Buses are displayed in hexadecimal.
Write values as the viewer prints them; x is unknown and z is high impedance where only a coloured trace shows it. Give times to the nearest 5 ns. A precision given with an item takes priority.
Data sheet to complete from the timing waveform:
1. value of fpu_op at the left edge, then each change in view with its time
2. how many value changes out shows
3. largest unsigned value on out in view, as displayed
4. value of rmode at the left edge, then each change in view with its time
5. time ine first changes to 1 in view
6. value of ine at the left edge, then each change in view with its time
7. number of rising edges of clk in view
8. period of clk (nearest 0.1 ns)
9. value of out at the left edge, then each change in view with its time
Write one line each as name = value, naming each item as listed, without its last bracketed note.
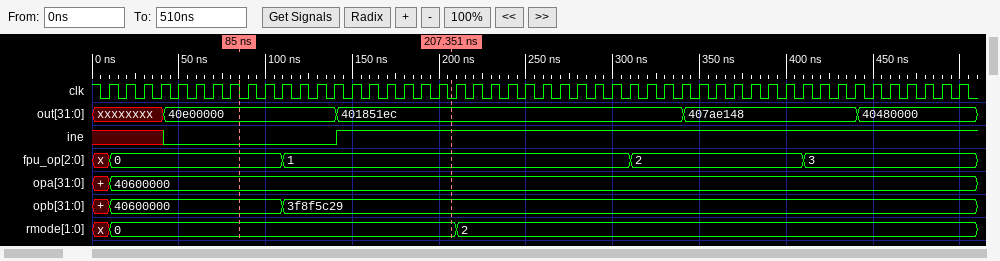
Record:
value of fpu_op at the left edge, then each change in view with its time = x, 0 at 10 ns, 1 at 110 ns, 2 at 310 ns, 3 at 410 ns
how many value changes out shows = 4
largest unsigned value on out in view, as displayed = 40e00000
value of rmode at the left edge, then each change in view with its time = x, 0 at 10 ns, 2 at 210 ns
time ine first changes to 1 in view = 140 ns
value of ine at the left edge, then each change in view with its time = x, 0 at 40 ns, 1 at 140 ns
number of rising edges of clk in view = 50
period of clk = 10 ns
value of out at the left edge, then each change in view with its time = xxxxxxxx, 40e00000 at 40 ns, 401851ec at 140 ns, 407ae148 at 340 ns, 40480000 at 440 ns
